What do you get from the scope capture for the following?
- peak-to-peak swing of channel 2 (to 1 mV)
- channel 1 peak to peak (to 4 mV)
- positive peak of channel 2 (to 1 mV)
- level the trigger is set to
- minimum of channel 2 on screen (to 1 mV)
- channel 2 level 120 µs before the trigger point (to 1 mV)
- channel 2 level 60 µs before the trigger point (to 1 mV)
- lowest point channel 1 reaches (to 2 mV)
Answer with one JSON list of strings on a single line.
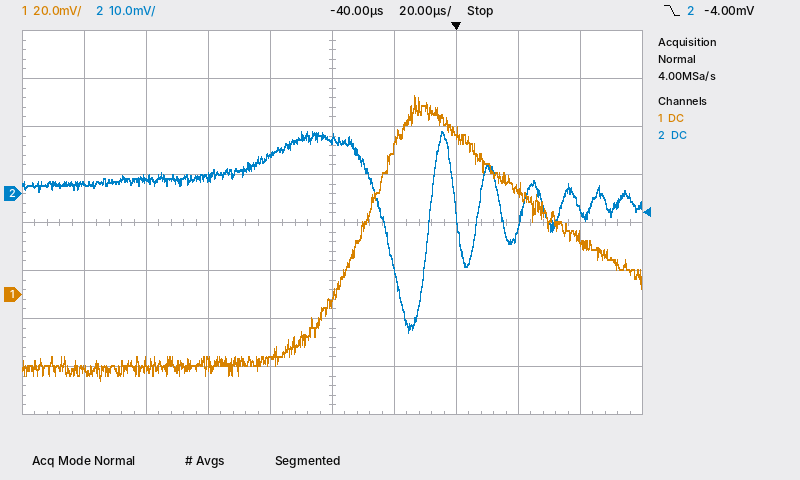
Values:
["42 mV", "120 mV", "13 mV", "-4.00 mV", "-29 mV", "2 mV", "8 mV", "-36 mV"]
